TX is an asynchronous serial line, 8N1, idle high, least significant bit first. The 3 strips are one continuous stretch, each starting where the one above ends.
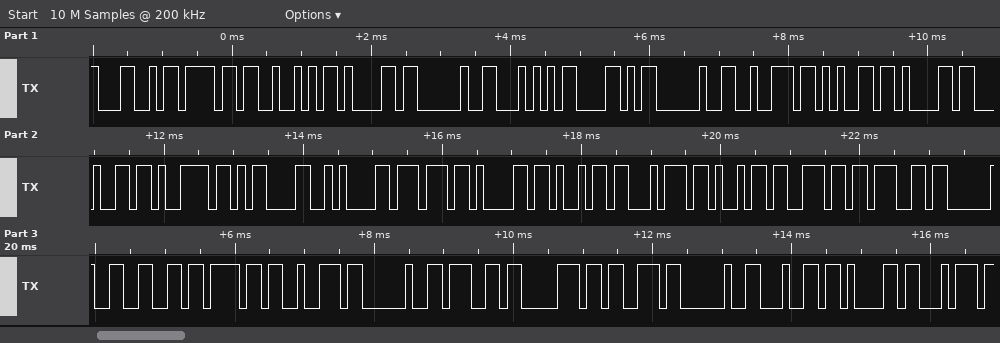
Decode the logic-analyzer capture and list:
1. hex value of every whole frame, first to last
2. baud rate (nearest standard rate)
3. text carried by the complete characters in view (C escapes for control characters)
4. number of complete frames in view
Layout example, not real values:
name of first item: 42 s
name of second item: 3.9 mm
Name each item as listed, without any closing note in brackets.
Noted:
hex value of every whole frame, first to last: 0x4C 0x6F 0x52 0x61 0x20 0x54 0x58 0x20 0x72 0x65 0x61 0x64 0x79 0x0D 0x0A 0x77 0x61 0x69 0x74 0x69 0x6E 0x67 0x20 0x66 0x6F 0x72 0x20 0x67 0x70 0x73 0x20 0x64 0x61 0x74
baud rate: 9600 baud
text carried by the complete characters in view: "LoRa TX ready\r\nwaiting for gps dat"
number of complete frames in view: 34
